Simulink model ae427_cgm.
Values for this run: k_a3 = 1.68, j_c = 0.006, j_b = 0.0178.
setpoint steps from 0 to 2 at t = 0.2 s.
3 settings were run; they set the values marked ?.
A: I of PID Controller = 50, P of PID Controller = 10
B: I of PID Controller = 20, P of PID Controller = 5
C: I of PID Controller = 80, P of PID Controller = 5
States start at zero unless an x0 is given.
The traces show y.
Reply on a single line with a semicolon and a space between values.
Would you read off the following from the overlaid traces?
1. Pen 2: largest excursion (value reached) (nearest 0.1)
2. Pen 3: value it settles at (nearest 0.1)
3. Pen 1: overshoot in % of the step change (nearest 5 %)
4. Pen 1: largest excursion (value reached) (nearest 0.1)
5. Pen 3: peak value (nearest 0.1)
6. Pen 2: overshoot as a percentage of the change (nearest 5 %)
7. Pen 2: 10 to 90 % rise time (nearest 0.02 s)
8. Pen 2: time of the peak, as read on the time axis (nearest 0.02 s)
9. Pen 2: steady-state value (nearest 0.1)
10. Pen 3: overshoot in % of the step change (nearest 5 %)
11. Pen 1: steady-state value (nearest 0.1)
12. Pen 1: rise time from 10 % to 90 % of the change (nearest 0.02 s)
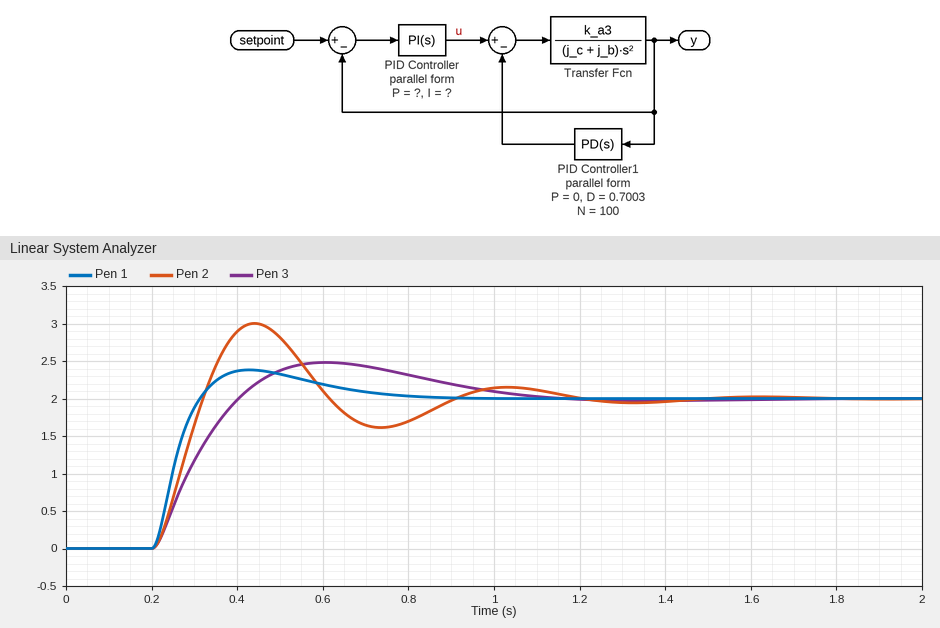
3.0; 2.0; 20 %; 2.4; 2.5; 50 %; 0.08 s; 0.44 s; 2.0; 25 %; 2.0; 0.08 s
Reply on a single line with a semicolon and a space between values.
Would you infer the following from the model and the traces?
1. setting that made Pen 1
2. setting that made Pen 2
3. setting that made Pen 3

A; C; B
